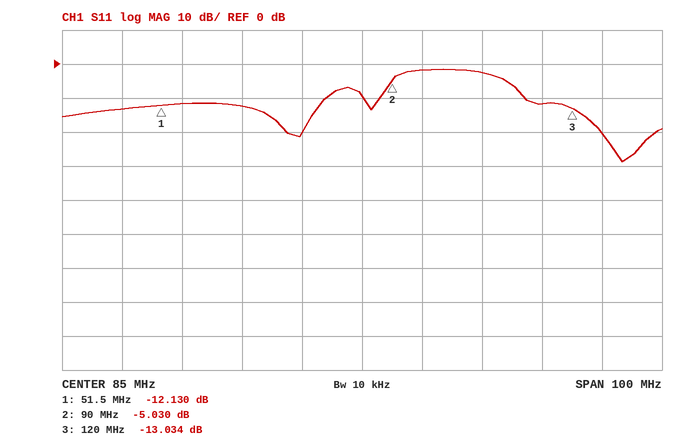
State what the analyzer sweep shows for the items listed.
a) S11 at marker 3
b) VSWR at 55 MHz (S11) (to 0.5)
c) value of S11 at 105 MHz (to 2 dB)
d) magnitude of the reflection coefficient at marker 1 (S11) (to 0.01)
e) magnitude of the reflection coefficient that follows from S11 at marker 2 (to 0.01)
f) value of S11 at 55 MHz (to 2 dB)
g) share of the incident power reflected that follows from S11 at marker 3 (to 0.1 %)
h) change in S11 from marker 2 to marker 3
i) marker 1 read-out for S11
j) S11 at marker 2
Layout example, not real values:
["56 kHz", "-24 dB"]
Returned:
["-13.034 dB", "1.5", "-2 dB", "0.25", "0.56", "-12 dB", "5.0 %", "-8.004 dB", "-12.130 dB", "-5.030 dB"]
